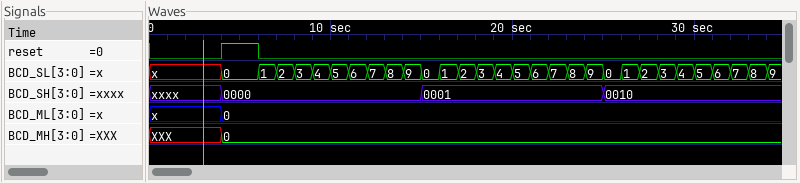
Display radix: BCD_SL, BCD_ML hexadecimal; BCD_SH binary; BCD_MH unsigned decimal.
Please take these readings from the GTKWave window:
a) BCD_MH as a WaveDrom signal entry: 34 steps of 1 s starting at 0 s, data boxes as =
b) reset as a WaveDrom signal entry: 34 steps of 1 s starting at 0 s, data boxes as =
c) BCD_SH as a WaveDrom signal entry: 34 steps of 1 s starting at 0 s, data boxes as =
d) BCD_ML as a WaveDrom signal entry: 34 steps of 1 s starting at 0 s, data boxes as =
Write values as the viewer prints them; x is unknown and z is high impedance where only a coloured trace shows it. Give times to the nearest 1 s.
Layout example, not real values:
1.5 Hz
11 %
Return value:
{name: 'BCD_MH', wave: 'x...=.............................', data: '0'}
{name: 'reset', wave: '0...1.0...........................'}
{name: 'BCD_SH', wave: 'x...=..........=.........=........', data: '0000 0001 0010'}
{name: 'BCD_ML', wave: 'x...=.............................', data: '0'}
